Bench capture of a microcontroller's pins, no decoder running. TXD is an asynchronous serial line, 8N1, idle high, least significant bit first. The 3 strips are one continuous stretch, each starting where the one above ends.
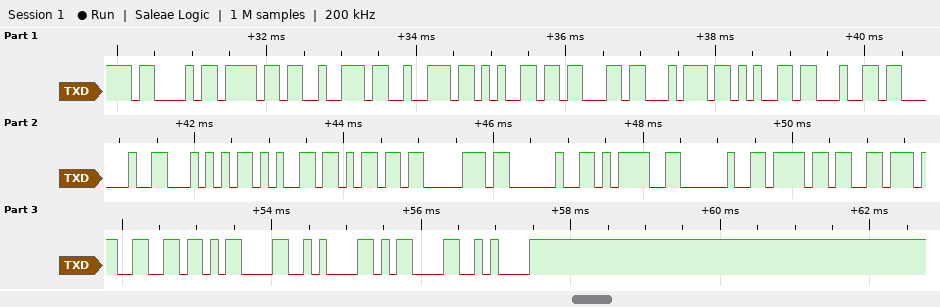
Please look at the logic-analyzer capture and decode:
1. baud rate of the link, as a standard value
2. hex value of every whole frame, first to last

9600 baud
43 6F 72 72 65 63 74 65 64 20 54 65 6D 70 20 3D 20 6F 76 66 0D 0A 0D 0A
